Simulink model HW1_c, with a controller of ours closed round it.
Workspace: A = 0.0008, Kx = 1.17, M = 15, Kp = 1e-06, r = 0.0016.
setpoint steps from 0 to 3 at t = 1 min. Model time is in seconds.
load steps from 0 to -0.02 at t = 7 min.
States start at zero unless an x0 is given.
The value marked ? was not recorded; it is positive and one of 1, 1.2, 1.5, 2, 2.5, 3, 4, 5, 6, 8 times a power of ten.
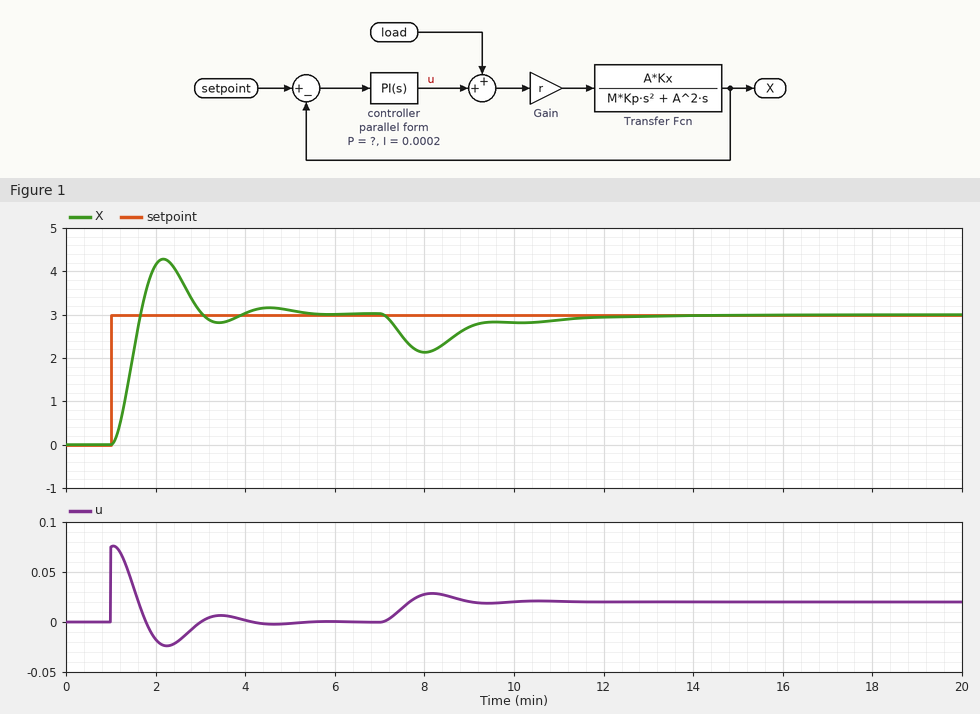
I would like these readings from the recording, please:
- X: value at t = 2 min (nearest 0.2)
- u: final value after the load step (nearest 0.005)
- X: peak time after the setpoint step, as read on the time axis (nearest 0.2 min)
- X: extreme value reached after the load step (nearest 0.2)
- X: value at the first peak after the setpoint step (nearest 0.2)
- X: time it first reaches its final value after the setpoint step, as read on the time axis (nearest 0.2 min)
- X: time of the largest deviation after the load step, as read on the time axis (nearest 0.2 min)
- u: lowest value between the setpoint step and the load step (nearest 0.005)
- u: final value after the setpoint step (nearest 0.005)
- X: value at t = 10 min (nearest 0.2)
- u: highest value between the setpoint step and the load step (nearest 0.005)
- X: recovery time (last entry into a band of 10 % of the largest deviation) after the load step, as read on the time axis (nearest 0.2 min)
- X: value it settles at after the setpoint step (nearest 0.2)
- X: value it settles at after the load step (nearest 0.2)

4.2
0.020
2.2 min
2.2
4.2
1.6 min
8.0 min
-0.025
0.000
2.8
0.075
11.4 min
3.0
3.0
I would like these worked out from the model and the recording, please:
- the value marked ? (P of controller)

0.025
